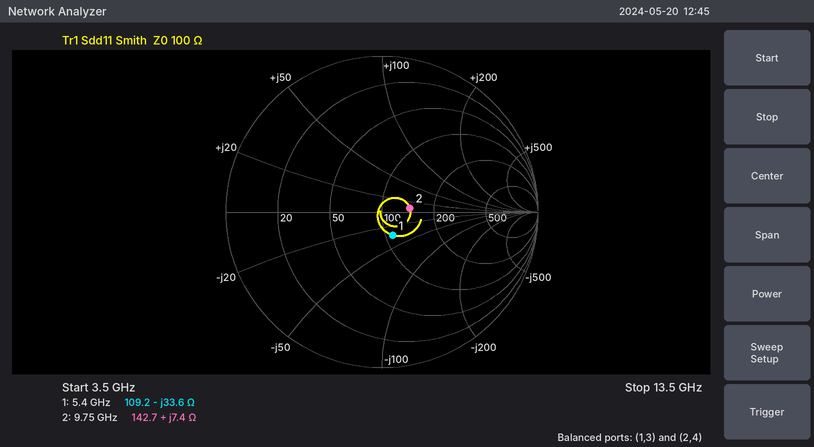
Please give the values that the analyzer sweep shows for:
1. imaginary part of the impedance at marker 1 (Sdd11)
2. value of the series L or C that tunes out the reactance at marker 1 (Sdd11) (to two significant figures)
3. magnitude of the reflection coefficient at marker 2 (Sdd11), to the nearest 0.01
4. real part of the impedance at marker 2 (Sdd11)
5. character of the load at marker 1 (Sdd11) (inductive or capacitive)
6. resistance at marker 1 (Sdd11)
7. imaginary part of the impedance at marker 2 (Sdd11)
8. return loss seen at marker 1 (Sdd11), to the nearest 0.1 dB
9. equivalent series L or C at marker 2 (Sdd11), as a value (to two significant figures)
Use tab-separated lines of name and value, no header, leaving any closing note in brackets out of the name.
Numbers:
imaginary part of the impedance at marker 1	-33.6 Ω
value of the series L or C that tunes out the reactance at marker 1 (Sdd11)	990 pH
magnitude of the reflection coefficient at marker 2 (Sdd11), to the nearest 0.01	0.18
real part of the impedance at marker 2	142.7 Ω
character of the load at marker 1 (Sdd11)	capacitive
resistance at marker 1	109.2 Ω
imaginary part of the impedance at marker 2	+7.4 Ω
return loss seen at marker 1 (Sdd11), to the nearest 0.1 dB	15.7 dB
equivalent series L or C at marker 2 (Sdd11), as a value	120 pH
